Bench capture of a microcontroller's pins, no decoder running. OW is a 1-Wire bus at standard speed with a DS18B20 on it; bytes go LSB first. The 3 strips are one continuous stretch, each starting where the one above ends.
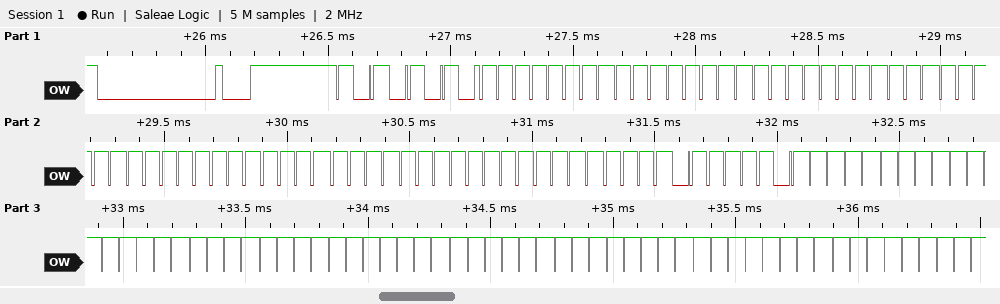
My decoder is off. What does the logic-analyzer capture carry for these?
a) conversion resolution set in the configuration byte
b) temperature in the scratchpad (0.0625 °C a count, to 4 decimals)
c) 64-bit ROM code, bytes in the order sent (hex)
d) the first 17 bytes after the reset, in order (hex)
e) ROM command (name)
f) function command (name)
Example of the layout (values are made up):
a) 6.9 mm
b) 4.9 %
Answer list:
a) 12 bits
b) -0.0625 °C
c) FF FF FF FF FF FF FF FF
d) 55 FF FF FF FF FF FF FF FF BE FF FF FF FF FF FF FF
e) Match ROM
f) Read Scratchpad
